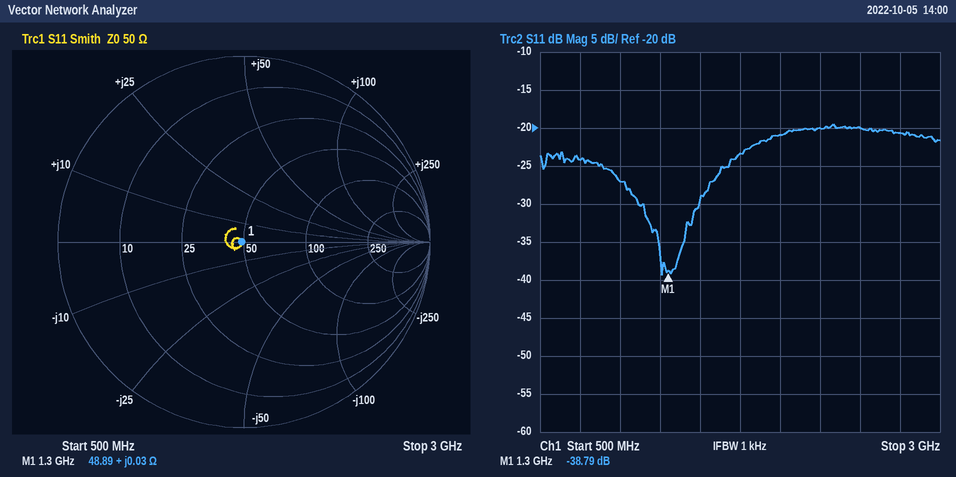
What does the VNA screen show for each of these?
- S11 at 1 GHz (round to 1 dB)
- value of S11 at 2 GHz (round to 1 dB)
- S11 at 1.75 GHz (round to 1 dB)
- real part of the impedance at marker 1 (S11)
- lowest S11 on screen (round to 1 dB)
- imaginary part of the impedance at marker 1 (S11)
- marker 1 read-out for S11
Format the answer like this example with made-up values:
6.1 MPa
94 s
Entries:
-27 dB
-21 dB
-23 dB
48.89 Ω
-39 dB
+0.03 Ω
-38.79 dB
